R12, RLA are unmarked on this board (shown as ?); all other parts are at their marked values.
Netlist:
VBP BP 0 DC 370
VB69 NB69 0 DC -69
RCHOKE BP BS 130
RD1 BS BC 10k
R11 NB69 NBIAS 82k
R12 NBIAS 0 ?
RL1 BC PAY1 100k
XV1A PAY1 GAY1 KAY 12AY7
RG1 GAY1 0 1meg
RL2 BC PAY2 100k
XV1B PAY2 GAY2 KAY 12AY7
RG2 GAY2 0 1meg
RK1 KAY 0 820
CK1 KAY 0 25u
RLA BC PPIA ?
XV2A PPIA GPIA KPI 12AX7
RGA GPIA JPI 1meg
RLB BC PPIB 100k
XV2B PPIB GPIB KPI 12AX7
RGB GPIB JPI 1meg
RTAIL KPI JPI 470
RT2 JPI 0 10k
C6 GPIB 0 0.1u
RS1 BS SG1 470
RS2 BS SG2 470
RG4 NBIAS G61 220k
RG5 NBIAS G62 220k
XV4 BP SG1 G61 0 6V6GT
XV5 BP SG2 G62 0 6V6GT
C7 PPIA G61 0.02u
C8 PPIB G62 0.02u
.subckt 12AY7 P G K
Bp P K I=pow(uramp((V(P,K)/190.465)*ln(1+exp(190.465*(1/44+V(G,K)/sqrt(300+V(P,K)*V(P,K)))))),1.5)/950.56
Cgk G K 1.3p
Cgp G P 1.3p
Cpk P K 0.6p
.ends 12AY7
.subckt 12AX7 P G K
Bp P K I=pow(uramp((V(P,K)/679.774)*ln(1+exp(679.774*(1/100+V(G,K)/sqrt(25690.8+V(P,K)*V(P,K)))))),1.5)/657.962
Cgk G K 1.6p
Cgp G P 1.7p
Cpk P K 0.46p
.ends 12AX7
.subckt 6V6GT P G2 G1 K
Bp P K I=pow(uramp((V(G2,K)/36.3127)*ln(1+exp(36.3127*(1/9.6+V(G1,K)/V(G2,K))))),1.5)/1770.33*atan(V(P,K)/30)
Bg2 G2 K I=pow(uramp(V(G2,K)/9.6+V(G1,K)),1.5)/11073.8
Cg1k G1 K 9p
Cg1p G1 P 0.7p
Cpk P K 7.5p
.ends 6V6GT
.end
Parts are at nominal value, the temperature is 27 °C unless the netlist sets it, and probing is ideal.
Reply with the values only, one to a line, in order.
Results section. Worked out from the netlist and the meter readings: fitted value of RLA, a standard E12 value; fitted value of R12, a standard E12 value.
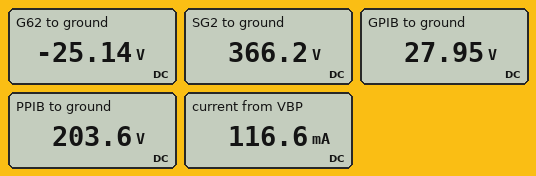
39 kΩ
47 kΩ
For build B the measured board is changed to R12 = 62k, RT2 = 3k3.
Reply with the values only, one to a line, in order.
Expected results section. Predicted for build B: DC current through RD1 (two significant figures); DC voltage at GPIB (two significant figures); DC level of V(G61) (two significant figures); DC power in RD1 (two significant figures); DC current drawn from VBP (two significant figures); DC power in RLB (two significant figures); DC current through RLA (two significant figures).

6.0 mA
9.8 V
-30 V
360 mW
82 mA
130 mW
1.8 mA
